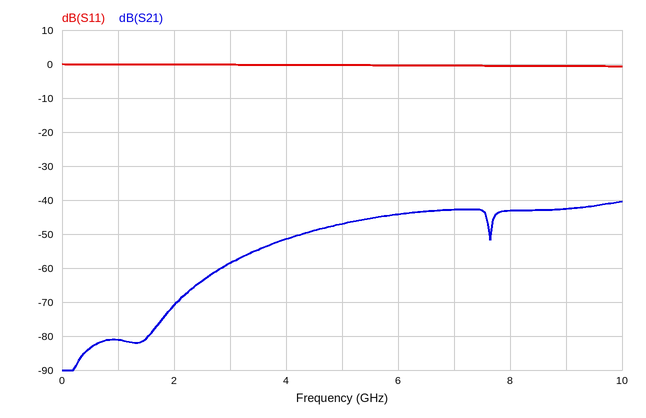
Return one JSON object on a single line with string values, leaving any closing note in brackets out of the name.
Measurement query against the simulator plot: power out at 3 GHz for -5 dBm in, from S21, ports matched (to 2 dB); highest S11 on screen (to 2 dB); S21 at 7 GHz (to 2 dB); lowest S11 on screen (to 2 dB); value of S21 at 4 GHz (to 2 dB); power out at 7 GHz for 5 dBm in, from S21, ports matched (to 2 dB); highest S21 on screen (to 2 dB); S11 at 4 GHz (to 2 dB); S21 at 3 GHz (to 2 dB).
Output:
{"power out at 3 GHz for -5 dBm in, from S21, ports matched": "-64 dBm", "highest S11 on screen": "0 dB", "S21 at 7 GHz": "-42 dB", "lowest S11 on screen": "0 dB", "value of S21 at 4 GHz": "-52 dB", "power out at 7 GHz for 5 dBm in, from S21, ports matched": "-38 dBm", "highest S21 on screen": "-40 dB", "S11 at 4 GHz": "0 dB", "S21 at 3 GHz": "-58 dB"}
